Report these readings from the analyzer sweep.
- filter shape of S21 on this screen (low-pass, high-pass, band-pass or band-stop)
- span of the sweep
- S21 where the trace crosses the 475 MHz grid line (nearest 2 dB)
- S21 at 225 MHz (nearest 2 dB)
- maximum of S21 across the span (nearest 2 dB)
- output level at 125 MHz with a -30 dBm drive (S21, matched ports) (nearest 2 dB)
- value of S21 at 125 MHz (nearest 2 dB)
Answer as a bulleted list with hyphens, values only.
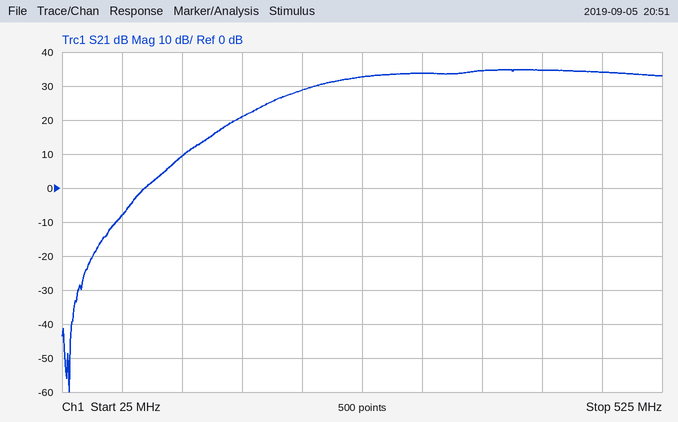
- high-pass
- 500 MHz
- 34 dB
- 28 dB
- 34 dB
- -20 dBm
- 10 dB
